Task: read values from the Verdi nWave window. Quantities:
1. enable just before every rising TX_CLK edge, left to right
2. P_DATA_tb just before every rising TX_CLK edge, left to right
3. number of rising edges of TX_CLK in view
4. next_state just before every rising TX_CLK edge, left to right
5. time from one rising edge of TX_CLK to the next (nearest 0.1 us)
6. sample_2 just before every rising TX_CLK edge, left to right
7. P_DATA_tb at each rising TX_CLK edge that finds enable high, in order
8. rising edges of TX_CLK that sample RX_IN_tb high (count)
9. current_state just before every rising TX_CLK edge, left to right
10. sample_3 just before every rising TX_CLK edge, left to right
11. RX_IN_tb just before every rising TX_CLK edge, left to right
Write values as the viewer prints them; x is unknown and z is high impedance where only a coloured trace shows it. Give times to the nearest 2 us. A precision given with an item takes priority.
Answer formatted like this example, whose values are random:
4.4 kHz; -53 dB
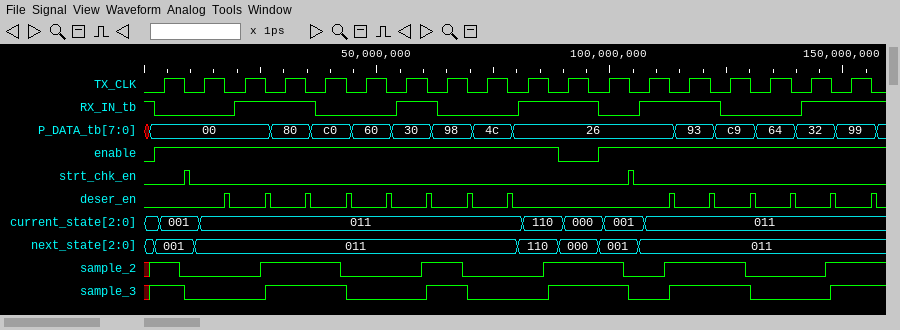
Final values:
1 1 1 1 1 1 1 1 1 1 0 1 1 1 1 1 1 1; 00, 00, 00, 80, c0, 60, 30, 98, 4c, 26, 26, 26, 26, 93, c9, 64, 32, 99; 18; 001, 011, 011, 011, 011, 011, 011, 011, 011, 110, 000, 001, 011, 011, 011, 011, 011, 011; 8.7 us; 1 0 0 1 1 0 0 1 0 0 1 1 0 1 1 0 0 1; 00, 00, 00, 80, c0, 60, 30, 98, 4c, 26, 26, 26, 93, c9, 64, 32, 99; 9; 001, 011, 011, 011, 011, 011, 011, 011, 011, 110, 000, 001, 011, 011, 011, 011, 011, 011; 1 0 0 1 1 0 0 1 0 0 1 1 0 1 1 0 0 1; 0 0 1 1 0 0 1 0 0 1 1 0 1 1 0 0 1 1
